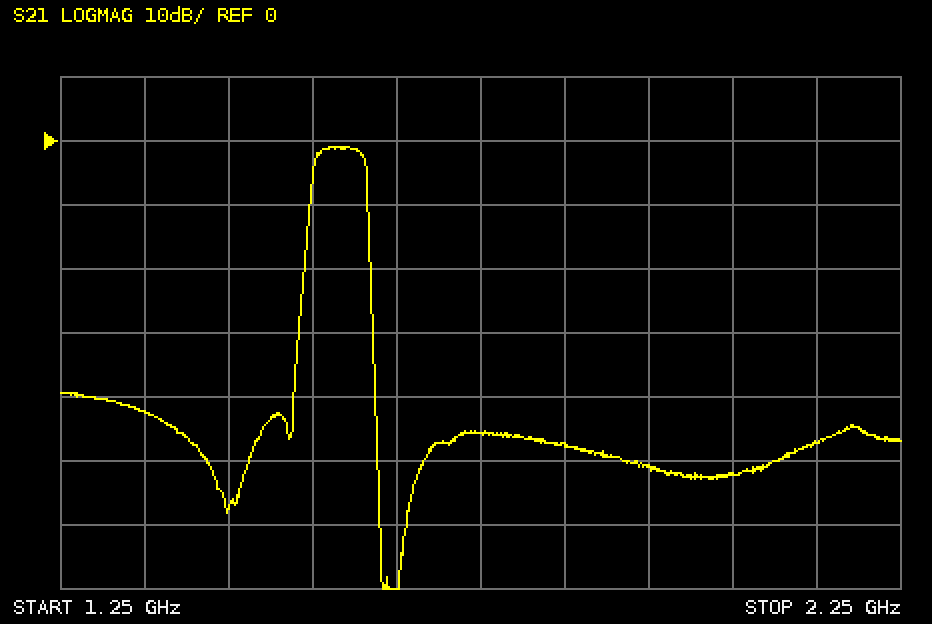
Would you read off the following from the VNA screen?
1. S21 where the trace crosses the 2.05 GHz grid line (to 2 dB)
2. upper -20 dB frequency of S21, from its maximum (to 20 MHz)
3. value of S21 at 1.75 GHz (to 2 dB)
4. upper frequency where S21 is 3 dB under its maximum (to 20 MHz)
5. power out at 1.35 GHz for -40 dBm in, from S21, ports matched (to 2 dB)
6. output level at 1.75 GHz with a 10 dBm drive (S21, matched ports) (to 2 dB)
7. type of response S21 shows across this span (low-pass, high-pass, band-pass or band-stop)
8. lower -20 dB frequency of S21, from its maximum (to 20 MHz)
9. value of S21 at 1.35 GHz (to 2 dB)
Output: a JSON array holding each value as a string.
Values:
["-52 dB", "1.62 GHz", "-46 dB", "1.62 GHz", "-82 dBm", "-36 dBm", "band-pass", "1.54 GHz", "-42 dB"]
